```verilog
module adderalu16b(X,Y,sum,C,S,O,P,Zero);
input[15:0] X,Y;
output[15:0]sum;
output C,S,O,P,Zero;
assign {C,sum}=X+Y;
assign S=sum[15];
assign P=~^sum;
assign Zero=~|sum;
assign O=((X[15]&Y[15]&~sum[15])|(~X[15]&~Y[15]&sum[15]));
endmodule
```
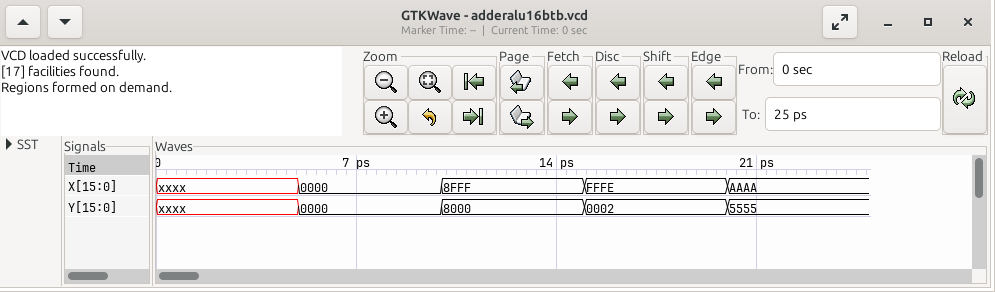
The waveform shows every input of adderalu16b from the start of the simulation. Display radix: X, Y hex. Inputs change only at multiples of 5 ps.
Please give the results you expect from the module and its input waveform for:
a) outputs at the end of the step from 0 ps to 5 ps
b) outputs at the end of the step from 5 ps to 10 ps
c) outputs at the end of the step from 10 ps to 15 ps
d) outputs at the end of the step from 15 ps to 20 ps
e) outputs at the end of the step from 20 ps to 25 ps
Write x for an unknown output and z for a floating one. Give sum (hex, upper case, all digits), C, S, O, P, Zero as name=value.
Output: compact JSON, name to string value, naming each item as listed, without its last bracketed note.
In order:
{"outputs at the end of the step from 0 ps to 5 ps": "sum=x, C=x, S=x, O=x, P=x, Zero=x", "outputs at the end of the step from 5 ps to 10 ps": "sum=0000, C=0, S=0, O=0, P=1, Zero=1", "outputs at the end of the step from 10 ps to 15 ps": "sum=0FFF, C=1, S=0, O=1, P=1, Zero=0", "outputs at the end of the step from 15 ps to 20 ps": "sum=0000, C=1, S=0, O=0, P=1, Zero=1", "outputs at the end of the step from 20 ps to 25 ps": "sum=FFFF, C=0, S=1, O=0, P=1, Zero=0"}
